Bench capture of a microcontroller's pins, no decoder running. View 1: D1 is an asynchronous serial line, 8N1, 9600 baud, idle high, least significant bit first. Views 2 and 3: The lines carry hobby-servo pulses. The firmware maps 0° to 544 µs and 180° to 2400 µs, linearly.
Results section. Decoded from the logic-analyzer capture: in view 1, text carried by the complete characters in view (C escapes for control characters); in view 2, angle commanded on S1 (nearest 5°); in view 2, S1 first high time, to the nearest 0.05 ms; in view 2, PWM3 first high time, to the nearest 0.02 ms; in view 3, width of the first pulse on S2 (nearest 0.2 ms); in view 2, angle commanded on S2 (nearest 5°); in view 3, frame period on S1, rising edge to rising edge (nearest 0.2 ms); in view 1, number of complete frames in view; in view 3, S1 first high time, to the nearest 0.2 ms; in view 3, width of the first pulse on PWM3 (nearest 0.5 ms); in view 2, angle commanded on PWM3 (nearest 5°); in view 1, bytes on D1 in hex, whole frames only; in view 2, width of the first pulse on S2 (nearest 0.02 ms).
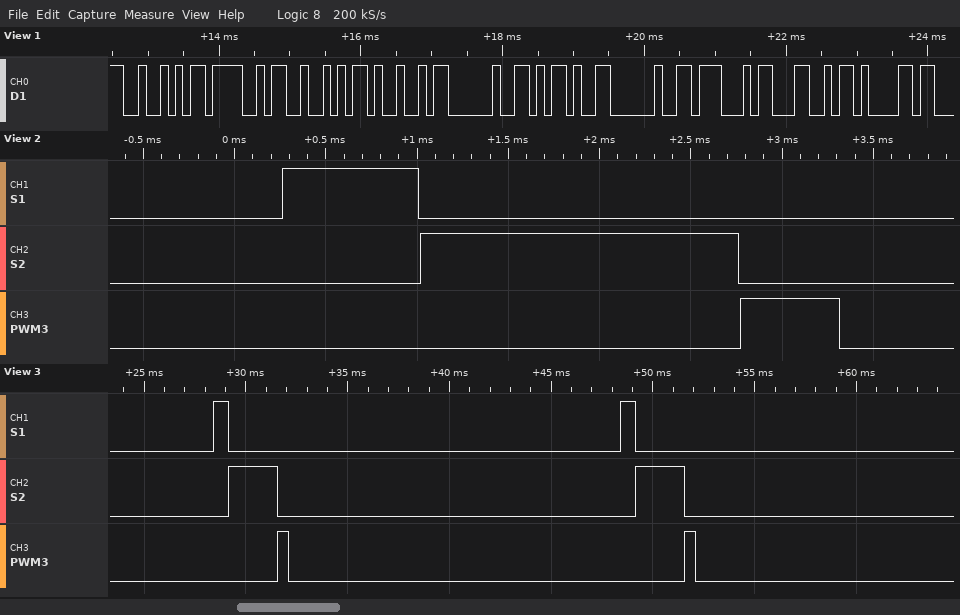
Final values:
"RORI - GLa"
20°
0.75 ms
0.54 ms
2.4 ms
115°
20.0 ms
10
0.8 ms
0.5 ms
0°
52 4F 52 49 20 2D 20 47 4C 61
1.74 ms
